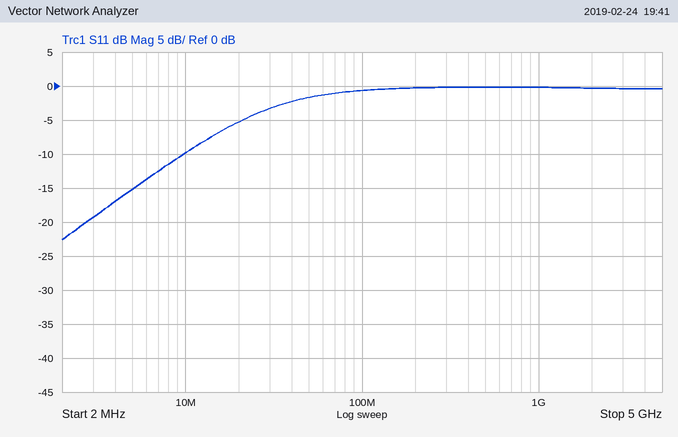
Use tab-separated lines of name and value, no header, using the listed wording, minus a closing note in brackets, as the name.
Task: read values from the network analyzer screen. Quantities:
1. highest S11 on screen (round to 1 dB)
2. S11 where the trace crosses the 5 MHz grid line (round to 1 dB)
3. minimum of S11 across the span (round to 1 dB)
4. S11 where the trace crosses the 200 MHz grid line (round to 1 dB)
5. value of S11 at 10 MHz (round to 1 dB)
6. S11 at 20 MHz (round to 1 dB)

highest S11 on screen	0 dB
S11 where the trace crosses the 5 MHz grid line	-15 dB
minimum of S11 across the span	-23 dB
S11 where the trace crosses the 200 MHz grid line	0 dB
value of S11 at 10 MHz	-10 dB
S11 at 20 MHz	-5 dB
